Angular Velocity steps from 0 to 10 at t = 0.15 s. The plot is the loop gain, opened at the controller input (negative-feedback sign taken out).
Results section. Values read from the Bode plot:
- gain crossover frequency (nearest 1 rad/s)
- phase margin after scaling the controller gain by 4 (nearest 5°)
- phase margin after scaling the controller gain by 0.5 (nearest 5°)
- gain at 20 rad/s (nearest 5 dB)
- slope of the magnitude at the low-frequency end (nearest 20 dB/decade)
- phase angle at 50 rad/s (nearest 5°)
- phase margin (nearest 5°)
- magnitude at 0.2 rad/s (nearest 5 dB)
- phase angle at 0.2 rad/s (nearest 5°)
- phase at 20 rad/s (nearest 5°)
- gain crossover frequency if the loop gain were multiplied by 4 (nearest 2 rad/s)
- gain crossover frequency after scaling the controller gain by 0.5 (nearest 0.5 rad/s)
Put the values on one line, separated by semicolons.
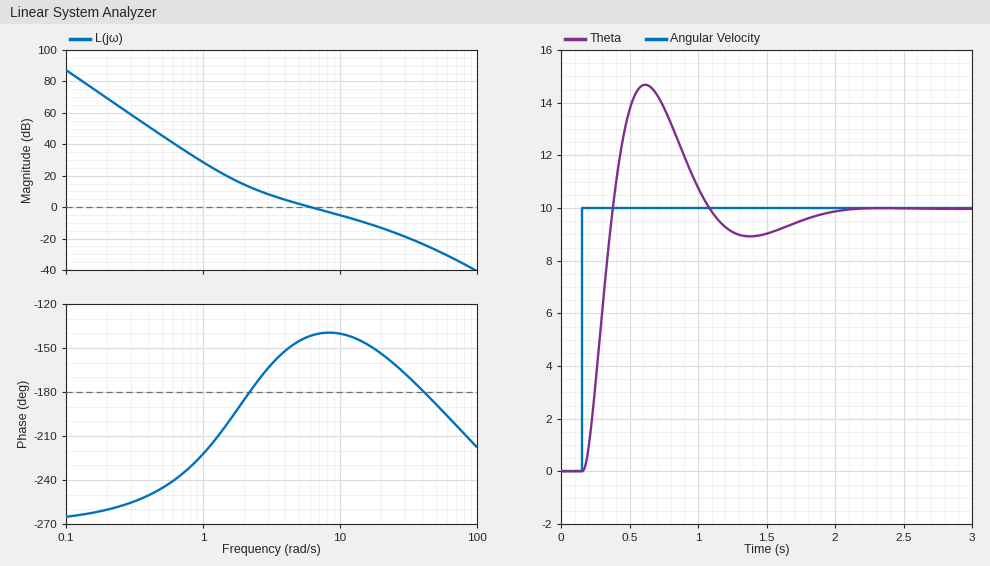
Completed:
6 rad/s; 30°; 25°; -15 dB; -60 dB/decade; -190°; 40°; 70 dB; -260°; -155°; 18 rad/s; 3.5 rad/s
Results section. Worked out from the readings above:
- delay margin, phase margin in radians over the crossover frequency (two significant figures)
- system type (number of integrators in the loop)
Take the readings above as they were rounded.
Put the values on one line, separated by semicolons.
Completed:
0.12 s; 3
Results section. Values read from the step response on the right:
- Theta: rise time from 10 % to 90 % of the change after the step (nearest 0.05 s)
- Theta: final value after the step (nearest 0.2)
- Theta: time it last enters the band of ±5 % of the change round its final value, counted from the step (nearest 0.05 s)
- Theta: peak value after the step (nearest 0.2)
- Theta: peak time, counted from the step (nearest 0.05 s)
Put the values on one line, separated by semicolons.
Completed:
0.15 s; 10.0; 1.60 s; 14.6; 0.45 s
